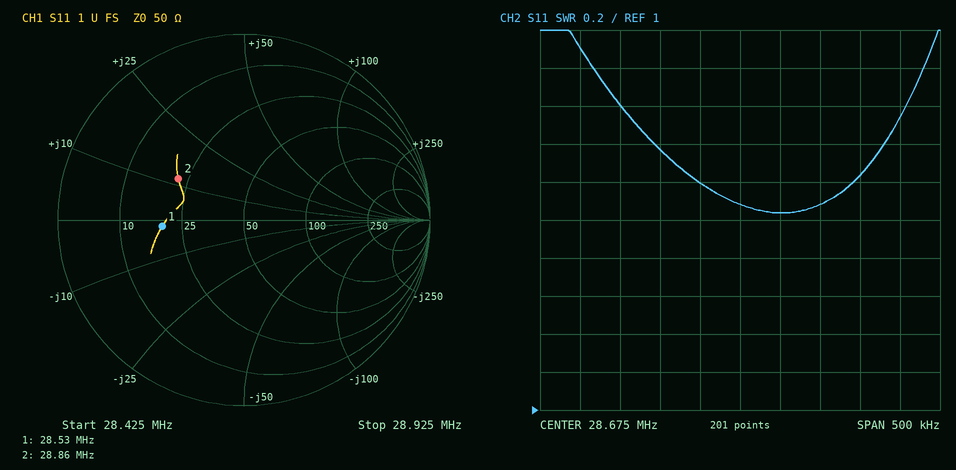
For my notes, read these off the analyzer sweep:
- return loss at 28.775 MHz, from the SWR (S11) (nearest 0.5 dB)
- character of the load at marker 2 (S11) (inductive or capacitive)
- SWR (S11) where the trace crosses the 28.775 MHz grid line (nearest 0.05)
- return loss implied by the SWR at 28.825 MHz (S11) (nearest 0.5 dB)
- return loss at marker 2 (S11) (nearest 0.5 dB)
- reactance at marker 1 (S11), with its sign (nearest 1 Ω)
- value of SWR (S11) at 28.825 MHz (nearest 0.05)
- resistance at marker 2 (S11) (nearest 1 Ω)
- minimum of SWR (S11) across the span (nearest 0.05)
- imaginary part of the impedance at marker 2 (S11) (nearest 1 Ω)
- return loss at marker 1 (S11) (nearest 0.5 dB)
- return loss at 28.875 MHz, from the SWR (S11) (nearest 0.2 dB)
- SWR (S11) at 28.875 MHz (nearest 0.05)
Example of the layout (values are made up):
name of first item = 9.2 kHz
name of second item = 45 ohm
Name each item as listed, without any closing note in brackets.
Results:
return loss at 28.775 MHz, from the SWR (S11) = 9.0 dB
character of the load at marker 2 (S11) = inductive
SWR (S11) where the trace crosses the 28.775 MHz grid line = 2.10
return loss implied by the SWR at 28.825 MHz (S11) = 8.5 dB
return loss at marker 2 (S11) = 7.5 dB
reactance at marker 1 (S11), with its sign = -2 Ω
value of SWR (S11) at 28.825 MHz = 2.25
resistance at marker 2 (S11) = 22 Ω
minimum of SWR (S11) across the span = 2.05
imaginary part of the impedance at marker 2 (S11) = +12 Ω
return loss at marker 1 (S11) = 7.0 dB
return loss at 28.875 MHz, from the SWR (S11) = 7.2 dB
SWR (S11) at 28.875 MHz = 2.55
